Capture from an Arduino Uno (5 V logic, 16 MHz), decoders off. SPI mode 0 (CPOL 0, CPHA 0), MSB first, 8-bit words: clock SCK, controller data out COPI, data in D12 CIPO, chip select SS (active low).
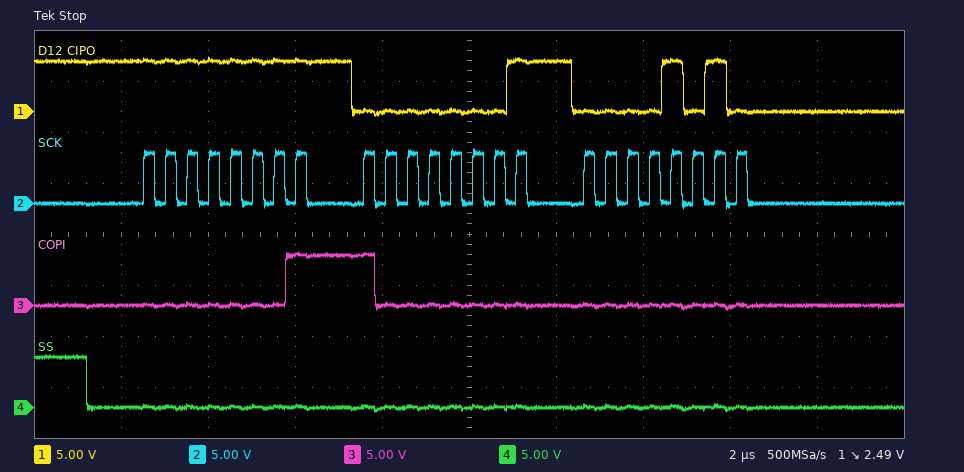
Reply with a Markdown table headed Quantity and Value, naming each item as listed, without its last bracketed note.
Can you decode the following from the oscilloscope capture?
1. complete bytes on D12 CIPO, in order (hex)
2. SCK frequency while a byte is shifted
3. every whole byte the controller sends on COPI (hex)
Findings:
| Quantity | Value |
|---|---|
| complete bytes on D12 CIPO, in order | FF 01 0A |
| SCK frequency while a byte is shifted | 2 MHz |
| every whole byte the controller sends on COPI | 01 80 00 |
